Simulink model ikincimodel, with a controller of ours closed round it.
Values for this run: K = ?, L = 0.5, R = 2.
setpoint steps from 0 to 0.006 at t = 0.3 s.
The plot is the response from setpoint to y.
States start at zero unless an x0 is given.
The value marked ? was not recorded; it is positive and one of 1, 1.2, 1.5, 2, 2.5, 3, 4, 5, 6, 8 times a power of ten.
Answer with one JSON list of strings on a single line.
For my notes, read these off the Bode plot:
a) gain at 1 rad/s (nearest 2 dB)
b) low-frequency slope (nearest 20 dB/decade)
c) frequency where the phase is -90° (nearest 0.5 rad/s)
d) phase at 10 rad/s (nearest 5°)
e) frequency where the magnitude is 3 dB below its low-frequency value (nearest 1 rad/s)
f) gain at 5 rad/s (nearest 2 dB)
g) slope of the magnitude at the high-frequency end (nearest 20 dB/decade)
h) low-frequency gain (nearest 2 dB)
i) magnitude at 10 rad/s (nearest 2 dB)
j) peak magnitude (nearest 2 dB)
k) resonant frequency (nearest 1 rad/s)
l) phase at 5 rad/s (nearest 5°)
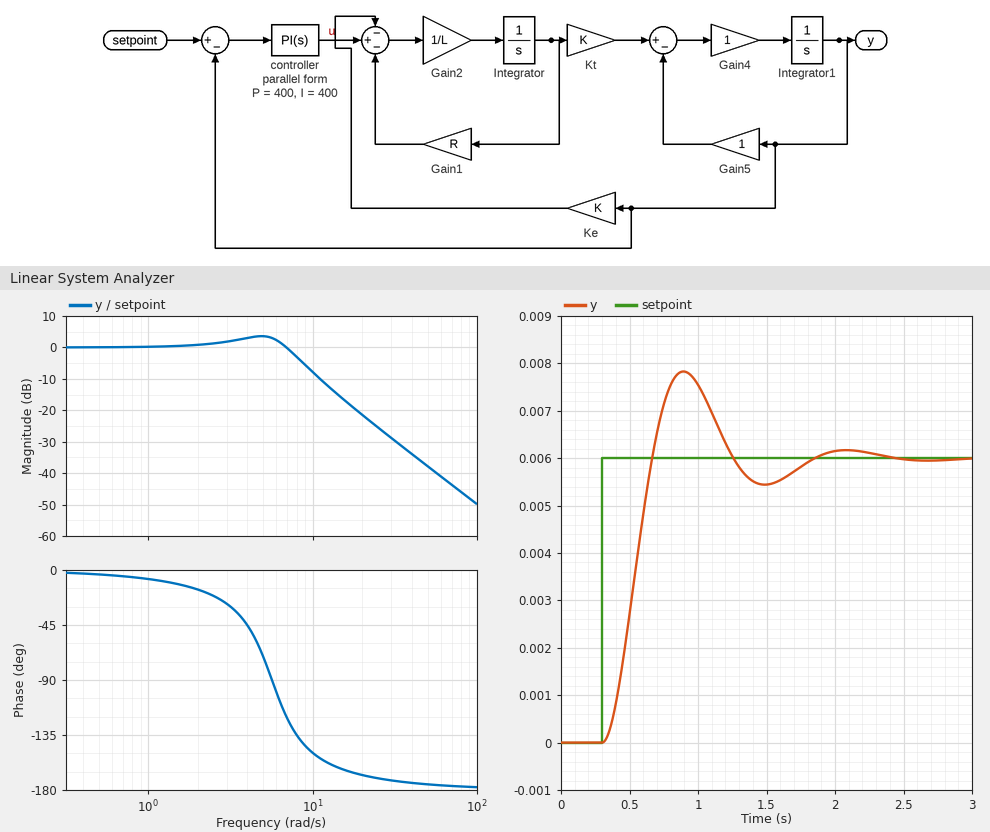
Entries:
["0 dB", "0 dB/decade", "5.5 rad/s", "-150°", "8 rad/s", "4 dB", "-40 dB/decade", "0 dB", "-8 dB", "4 dB", "5 rad/s", "-70°"]
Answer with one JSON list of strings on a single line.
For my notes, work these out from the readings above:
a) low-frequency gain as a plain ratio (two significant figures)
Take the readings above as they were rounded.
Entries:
["1.0"]
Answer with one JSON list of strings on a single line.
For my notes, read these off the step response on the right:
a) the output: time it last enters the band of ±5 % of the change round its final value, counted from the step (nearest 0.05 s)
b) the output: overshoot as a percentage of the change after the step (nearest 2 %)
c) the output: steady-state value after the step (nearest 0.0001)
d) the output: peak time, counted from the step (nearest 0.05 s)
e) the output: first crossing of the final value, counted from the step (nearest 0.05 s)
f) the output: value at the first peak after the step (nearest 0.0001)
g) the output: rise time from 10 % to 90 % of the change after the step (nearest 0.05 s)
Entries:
["1.40 s", "30 %", "0.0060", "0.60 s", "0.35 s", "0.0078", "0.25 s"]
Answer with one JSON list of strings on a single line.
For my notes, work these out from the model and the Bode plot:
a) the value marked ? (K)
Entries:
["0.04"]
